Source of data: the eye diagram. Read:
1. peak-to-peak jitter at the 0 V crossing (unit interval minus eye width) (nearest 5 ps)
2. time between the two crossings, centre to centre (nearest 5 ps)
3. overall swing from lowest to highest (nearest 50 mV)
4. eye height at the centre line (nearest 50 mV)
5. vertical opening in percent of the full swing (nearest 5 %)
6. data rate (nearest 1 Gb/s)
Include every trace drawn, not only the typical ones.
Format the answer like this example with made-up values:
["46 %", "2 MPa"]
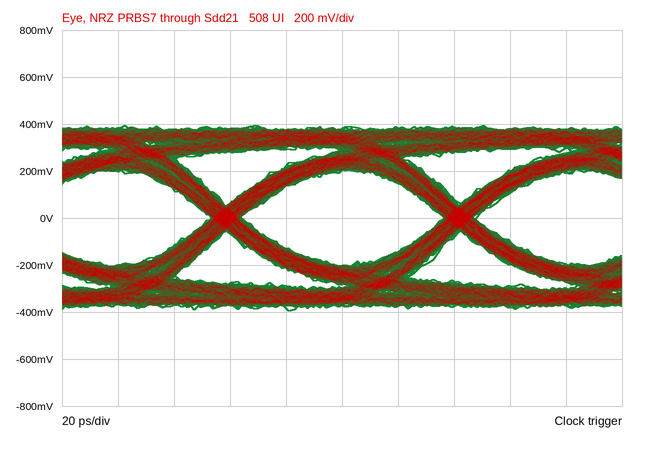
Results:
["10 ps", "85 ps", "800 mV", "400 mV", "50 %", "12 Gb/s"]
